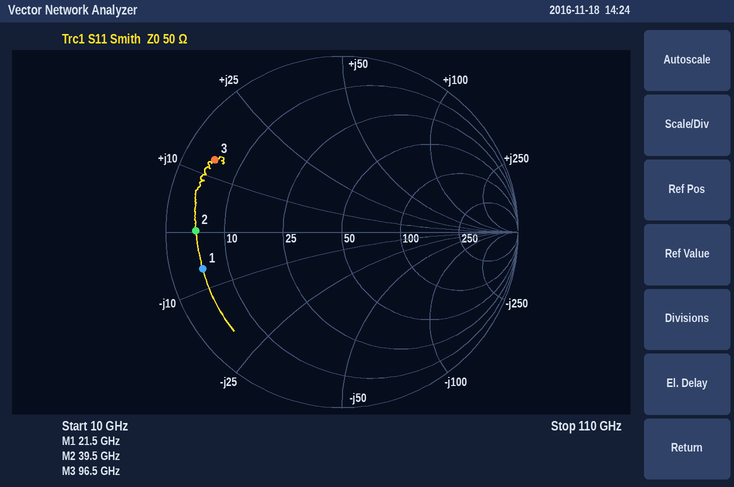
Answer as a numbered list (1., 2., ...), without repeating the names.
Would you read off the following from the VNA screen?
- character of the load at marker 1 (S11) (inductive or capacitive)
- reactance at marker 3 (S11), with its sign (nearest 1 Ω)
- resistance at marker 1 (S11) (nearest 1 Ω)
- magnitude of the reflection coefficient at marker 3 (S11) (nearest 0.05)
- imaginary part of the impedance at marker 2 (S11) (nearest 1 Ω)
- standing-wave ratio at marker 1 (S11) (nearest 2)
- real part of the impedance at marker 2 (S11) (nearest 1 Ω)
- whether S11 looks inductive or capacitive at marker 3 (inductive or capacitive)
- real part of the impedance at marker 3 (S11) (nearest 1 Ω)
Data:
1. capacitive
2. +13 Ω
3. 5 Ω
4. 0.85
5. 0 Ω
6. 10
7. 5 Ω
8. inductive
9. 5 Ω
